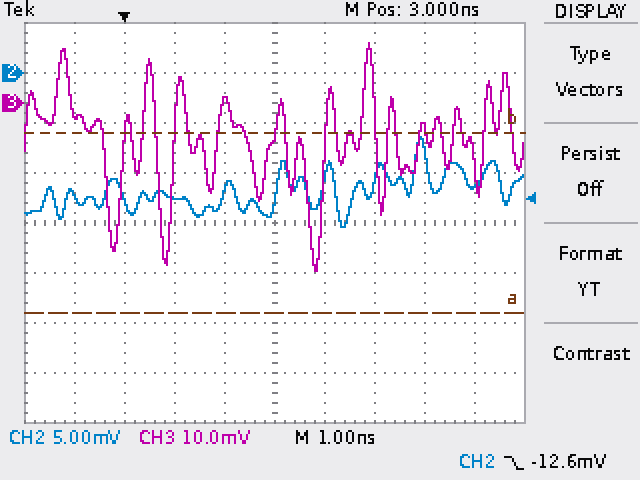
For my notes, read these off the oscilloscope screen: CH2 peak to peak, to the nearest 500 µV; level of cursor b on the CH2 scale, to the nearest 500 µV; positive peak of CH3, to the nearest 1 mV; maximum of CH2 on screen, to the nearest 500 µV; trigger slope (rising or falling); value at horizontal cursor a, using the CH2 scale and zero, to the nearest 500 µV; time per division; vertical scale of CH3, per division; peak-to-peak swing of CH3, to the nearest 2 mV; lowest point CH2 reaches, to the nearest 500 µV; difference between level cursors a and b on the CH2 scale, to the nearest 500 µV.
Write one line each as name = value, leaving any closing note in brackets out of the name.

CH2 peak to peak, to the nearest 500 µV = 9.0 mV
level of cursor b on the CH2 scale, to the nearest 500 µV = -6.0 mV
positive peak of CH3, to the nearest 1 mV = 12 mV
maximum of CH2 on screen, to the nearest 500 µV = -6.5 mV
trigger slope = falling
value at horizontal cursor a, using the CH2 scale and zero, to the nearest 500 µV = -24.0 mV
time per division = 1 ns
vertical scale of CH3, per division = 10 mV
peak-to-peak swing of CH3, to the nearest 2 mV = 46 mV
lowest point CH2 reaches, to the nearest 500 µV = -15.5 mV
difference between level cursors a and b on the CH2 scale, to the nearest 500 µV = 18.0 mV
